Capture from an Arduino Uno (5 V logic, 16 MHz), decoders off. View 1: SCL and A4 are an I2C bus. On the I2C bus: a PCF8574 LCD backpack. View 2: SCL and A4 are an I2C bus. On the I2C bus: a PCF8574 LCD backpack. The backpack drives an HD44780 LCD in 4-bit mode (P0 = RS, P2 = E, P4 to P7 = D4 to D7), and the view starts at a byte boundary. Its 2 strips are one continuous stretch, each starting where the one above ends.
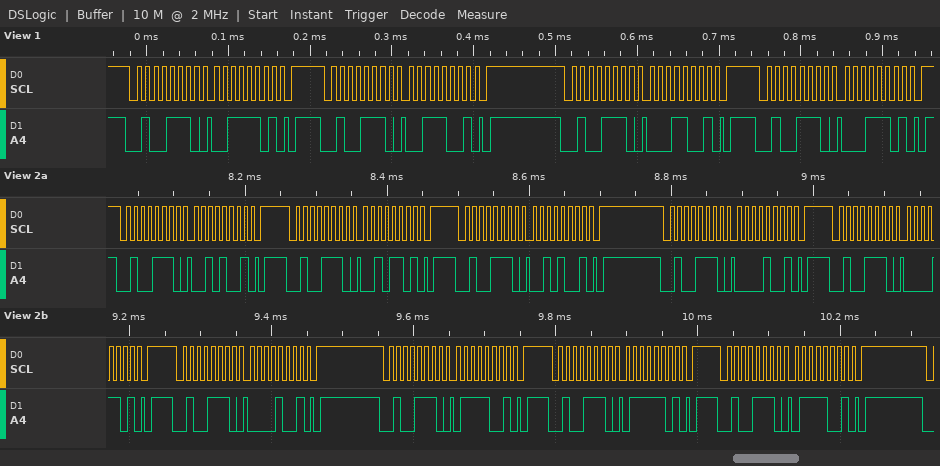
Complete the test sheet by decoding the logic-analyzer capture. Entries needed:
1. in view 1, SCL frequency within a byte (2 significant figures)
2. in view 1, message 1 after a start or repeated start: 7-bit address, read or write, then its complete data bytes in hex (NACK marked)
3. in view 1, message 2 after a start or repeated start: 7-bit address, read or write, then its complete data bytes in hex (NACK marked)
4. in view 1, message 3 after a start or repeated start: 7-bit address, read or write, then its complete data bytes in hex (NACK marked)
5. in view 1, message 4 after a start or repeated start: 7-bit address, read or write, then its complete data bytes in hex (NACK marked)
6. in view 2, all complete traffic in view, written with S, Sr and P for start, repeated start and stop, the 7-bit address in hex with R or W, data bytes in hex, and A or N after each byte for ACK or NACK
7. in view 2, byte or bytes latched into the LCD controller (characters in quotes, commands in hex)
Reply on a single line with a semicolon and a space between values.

100 kHz; 0x27 write: 3D; 0x27 write: 39; 0x27 write: 19; 0x27 write: 1D; S 27W A 29 A P S 27W A 2D A P S 27W A 29 A P S 27W A 09 A P S 27W A 0D A P S 27W A 09 A P S 27W A 79 A P S 27W A 7D A P S 27W A 79 A P; ' '
